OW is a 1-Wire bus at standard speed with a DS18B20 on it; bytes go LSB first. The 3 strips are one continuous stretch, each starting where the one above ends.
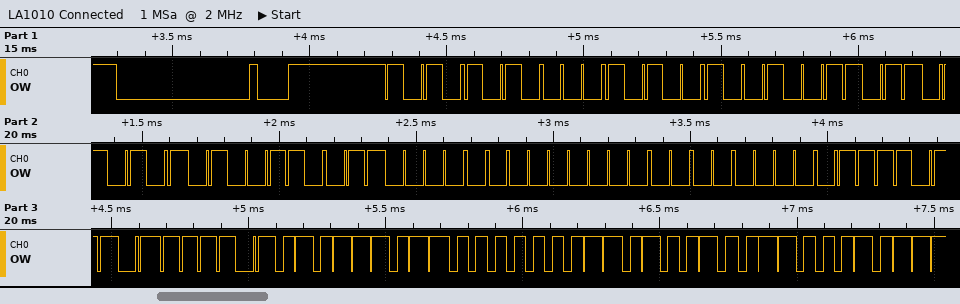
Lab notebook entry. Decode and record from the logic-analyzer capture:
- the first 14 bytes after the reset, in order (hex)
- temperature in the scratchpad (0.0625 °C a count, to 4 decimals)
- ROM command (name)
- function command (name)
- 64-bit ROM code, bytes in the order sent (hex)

55 28 C9 56 65 06 00 00 DE BE BA 01 4B 46
27.6250 °C
Match ROM
Read Scratchpad
28 C9 56 65 06 00 00 DE
